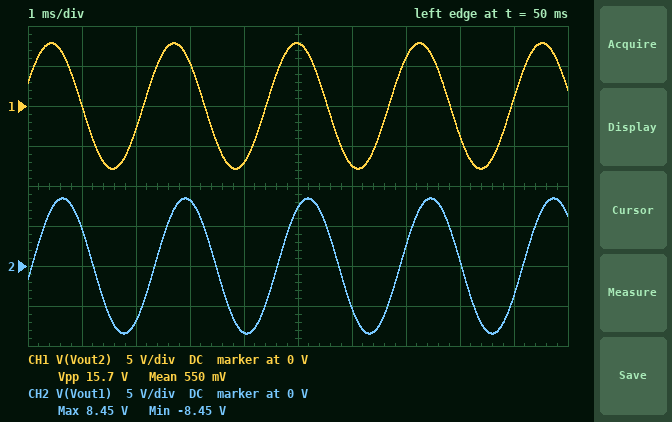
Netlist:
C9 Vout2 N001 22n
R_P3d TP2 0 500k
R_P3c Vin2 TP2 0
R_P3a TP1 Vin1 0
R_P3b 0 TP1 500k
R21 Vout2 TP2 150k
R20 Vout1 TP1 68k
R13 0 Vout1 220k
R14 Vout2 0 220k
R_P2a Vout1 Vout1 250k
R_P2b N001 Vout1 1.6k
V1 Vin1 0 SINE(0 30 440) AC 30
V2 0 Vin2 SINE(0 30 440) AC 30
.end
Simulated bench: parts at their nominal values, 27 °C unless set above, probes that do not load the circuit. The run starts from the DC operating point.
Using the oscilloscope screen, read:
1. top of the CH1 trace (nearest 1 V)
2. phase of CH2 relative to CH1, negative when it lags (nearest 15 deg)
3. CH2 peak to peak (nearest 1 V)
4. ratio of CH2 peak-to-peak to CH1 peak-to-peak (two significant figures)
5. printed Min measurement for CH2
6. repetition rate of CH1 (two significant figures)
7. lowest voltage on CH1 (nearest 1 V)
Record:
8 V
-30 deg
17 V
1.1
-8.45 V
440 Hz
-8 V
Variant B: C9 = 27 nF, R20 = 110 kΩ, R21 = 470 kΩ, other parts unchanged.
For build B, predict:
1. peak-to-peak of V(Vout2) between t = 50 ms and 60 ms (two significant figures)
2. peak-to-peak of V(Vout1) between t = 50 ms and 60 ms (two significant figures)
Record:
20 V
21 V
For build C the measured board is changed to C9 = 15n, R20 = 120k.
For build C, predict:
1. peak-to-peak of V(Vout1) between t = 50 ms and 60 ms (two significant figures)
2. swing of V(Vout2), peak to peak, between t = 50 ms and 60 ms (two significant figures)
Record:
7.1 V
6.3 V
